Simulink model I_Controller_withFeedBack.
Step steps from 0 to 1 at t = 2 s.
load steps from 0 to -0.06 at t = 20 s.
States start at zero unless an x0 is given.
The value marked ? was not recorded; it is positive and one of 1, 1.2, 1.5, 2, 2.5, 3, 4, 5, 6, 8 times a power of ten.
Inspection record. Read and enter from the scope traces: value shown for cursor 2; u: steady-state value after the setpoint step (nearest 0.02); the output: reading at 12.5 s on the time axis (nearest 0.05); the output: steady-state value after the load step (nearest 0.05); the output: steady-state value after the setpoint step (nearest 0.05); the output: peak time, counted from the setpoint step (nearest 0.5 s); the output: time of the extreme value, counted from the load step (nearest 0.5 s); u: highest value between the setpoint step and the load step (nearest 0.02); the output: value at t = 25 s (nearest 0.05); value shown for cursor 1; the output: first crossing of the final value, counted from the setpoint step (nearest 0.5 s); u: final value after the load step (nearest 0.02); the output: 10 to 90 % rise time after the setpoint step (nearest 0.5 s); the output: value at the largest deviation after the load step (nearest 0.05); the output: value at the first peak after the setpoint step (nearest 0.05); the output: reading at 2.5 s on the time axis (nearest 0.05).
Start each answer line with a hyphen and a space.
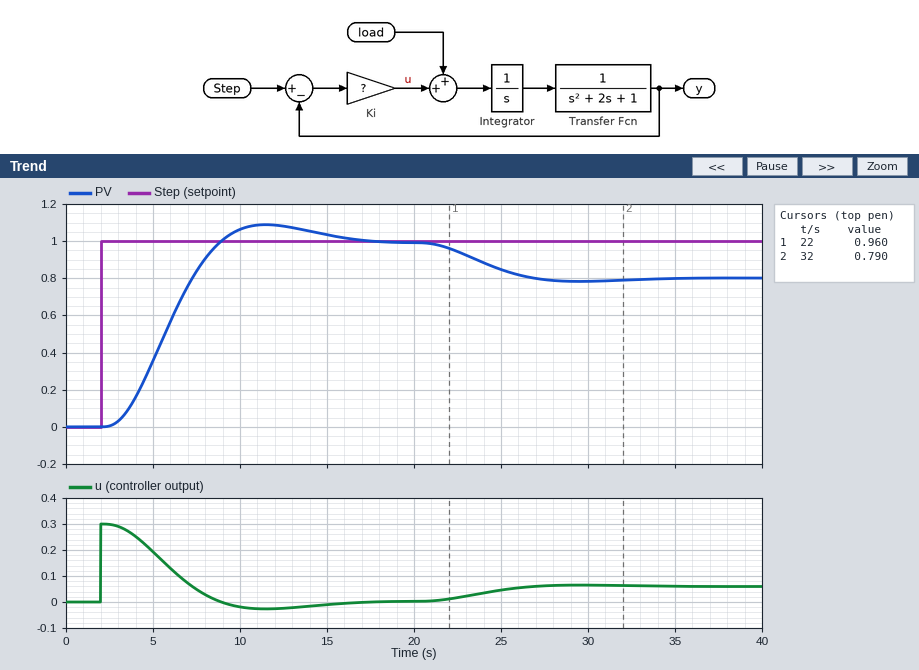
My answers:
- 0.790
- 0.00
- 1.10
- 0.80
- 1.00
- 9.5 s
- 9.5 s
- 0.30
- 0.85
- 0.960
- 7.0 s
- 0.06
- 4.5 s
- 0.80
- 1.10
- 0.00
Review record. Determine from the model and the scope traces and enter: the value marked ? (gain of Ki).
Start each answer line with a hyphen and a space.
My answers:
- 0.3
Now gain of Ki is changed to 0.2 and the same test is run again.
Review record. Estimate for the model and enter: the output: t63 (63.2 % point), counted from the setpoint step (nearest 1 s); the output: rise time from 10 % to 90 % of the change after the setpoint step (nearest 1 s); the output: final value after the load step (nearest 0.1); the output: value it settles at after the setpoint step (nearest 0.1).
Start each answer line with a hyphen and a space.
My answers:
- 6 s
- 7 s
- 0.7
- 1.0
